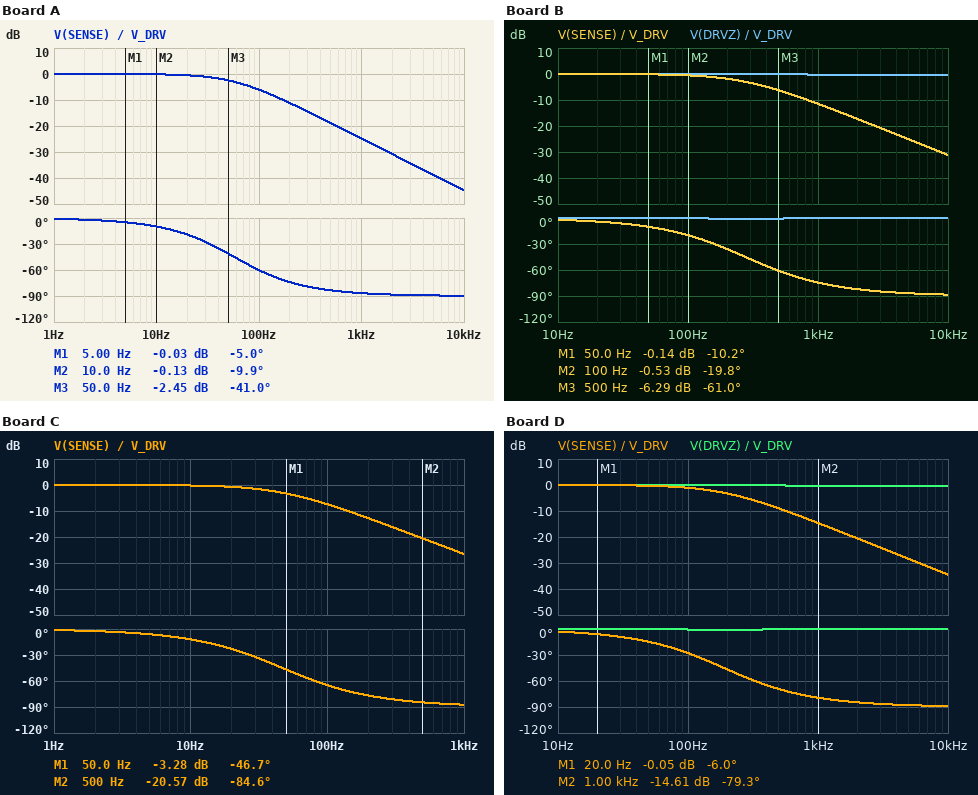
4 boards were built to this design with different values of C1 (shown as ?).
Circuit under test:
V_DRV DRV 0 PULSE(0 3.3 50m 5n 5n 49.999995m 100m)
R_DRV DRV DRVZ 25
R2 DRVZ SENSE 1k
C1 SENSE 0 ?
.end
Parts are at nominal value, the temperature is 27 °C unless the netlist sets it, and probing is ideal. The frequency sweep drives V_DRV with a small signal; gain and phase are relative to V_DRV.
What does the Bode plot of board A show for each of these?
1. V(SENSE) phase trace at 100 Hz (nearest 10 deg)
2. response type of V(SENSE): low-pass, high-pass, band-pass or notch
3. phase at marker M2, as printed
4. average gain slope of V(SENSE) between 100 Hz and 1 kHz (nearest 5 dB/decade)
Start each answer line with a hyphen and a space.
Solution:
- -60 deg
- low-pass
- -9.9 deg
- -20 dB/decade
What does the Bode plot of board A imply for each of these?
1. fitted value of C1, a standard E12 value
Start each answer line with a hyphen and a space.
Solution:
- 2.7 µF
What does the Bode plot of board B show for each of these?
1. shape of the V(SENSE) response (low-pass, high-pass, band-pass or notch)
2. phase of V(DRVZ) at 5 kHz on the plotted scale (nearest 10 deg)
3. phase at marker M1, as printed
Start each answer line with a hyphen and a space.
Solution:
- low-pass
- 0 deg
- -10.2 deg
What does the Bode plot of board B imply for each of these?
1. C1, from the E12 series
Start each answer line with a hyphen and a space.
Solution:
- 560 nF
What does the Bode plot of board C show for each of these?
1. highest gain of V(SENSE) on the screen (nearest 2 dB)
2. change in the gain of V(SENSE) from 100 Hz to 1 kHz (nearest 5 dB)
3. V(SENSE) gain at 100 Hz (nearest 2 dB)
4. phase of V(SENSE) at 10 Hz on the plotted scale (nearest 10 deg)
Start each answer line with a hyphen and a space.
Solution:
- 0 dB
- -20 dB
- -8 dB
- -10 deg
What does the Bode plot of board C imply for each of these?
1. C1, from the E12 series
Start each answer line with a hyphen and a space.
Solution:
- 3.3 µF
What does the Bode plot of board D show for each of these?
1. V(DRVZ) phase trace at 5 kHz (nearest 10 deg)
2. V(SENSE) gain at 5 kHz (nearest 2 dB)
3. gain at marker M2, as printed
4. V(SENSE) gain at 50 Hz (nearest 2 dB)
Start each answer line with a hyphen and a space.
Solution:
- 0 deg
- -28 dB
- -14.61 dB
- 0 dB
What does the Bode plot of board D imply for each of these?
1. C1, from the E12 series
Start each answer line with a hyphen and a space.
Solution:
- 820 nF
